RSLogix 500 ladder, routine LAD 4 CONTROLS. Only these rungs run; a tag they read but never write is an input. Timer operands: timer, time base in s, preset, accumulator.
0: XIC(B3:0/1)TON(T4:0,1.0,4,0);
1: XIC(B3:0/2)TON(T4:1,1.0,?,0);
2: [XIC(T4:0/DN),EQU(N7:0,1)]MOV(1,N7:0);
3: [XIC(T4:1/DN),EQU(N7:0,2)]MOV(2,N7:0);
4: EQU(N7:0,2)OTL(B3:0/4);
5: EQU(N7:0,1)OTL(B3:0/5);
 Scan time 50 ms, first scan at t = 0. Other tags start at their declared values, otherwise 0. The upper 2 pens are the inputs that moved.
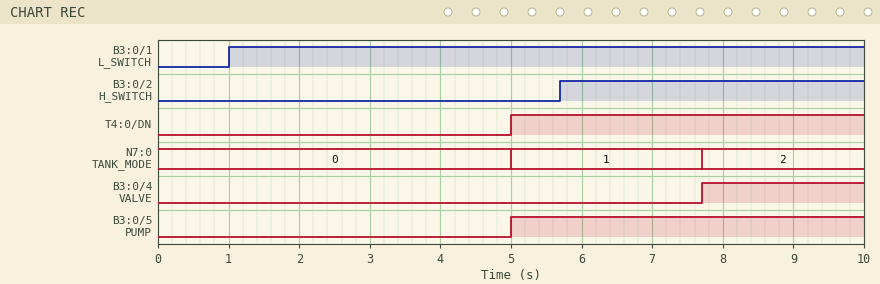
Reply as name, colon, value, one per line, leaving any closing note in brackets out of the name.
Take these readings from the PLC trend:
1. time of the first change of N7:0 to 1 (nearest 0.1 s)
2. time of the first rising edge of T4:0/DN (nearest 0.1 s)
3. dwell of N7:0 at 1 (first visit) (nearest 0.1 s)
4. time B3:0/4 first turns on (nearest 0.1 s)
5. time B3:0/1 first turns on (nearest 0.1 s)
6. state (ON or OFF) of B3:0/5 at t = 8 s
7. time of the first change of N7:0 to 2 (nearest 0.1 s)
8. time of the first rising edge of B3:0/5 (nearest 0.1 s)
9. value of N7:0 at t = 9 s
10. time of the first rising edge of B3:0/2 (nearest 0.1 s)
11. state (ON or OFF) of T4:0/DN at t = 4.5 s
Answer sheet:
time of the first change of N7:0 to 1: 5.0 s
time of the first rising edge of T4:0/DN: 5.0 s
dwell of N7:0 at 1 (first visit): 2.7 s
time B3:0/4 first turns on: 7.7 s
time B3:0/1 first turns on: 1.0 s
state (ON or OFF) of B3:0/5 at t = 8 s: ON
time of the first change of N7:0 to 2: 7.7 s
time of the first rising edge of B3:0/5: 5.0 s
value of N7:0 at t = 9 s: 2
time of the first rising edge of B3:0/2: 5.7 s
state (ON or OFF) of T4:0/DN at t = 4.5 s: OFF
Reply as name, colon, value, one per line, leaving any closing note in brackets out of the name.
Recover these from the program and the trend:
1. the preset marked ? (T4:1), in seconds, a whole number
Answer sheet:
the preset marked ? (T4:1), in seconds, a whole number: 2 s
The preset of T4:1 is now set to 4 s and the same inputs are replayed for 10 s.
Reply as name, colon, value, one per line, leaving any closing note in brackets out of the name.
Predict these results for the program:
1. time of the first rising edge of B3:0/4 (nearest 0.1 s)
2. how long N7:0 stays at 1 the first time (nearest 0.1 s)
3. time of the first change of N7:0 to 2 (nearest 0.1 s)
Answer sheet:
time of the first rising edge of B3:0/4: 9.7 s
how long N7:0 stays at 1 the first time: 4.7 s
time of the first change of N7:0 to 2: 9.7 s
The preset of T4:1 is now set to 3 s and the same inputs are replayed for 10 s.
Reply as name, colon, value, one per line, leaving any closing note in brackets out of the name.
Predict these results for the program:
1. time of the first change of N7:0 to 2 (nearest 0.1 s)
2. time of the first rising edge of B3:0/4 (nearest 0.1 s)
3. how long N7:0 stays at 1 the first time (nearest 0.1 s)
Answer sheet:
time of the first change of N7:0 to 2: 8.7 s
time of the first rising edge of B3:0/4: 8.7 s
how long N7:0 stays at 1 the first time: 3.7 s
